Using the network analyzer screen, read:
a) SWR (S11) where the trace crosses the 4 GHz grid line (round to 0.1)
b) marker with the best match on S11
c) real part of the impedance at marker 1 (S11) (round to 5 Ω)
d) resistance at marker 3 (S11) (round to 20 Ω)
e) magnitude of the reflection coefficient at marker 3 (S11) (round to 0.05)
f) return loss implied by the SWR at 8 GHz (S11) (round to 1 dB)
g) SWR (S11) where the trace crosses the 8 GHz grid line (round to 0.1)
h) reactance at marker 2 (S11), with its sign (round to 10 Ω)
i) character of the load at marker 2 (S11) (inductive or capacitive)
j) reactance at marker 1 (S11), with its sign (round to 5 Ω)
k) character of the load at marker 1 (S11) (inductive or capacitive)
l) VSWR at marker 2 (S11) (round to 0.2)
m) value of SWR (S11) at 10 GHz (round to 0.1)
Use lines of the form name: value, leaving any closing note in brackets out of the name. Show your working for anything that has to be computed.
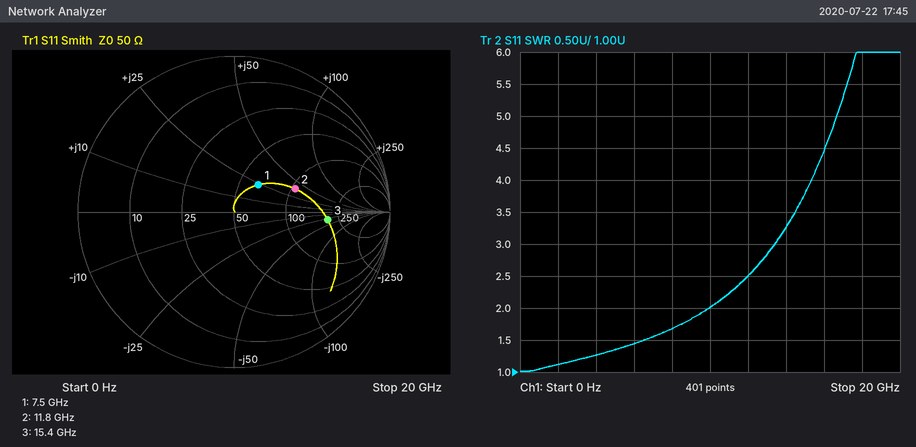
SWR (S11) where the trace crosses the 4 GHz grid line: 1.3
marker with the best match on S11: marker 1
real part of the impedance at marker 1 (S11): 65 Ω
resistance at marker 3 (S11): 200 Ω
magnitude of the reflection coefficient at marker 3 (S11): 0.60
return loss implied by the SWR at 8 GHz (S11): −20 log10((1.7 − 1)/(1.7 + 1)) ≈ 12 dB
SWR (S11) where the trace crosses the 8 GHz grid line: 1.7
reactance at marker 2 (S11), with its sign: +40 Ω
character of the load at marker 2 (S11): inductive
reactance at marker 1 (S11), with its sign: +25 Ω
character of the load at marker 1 (S11): inductive
VSWR at marker 2 (S11): 2.4
value of SWR (S11) at 10 GHz: 2.0
